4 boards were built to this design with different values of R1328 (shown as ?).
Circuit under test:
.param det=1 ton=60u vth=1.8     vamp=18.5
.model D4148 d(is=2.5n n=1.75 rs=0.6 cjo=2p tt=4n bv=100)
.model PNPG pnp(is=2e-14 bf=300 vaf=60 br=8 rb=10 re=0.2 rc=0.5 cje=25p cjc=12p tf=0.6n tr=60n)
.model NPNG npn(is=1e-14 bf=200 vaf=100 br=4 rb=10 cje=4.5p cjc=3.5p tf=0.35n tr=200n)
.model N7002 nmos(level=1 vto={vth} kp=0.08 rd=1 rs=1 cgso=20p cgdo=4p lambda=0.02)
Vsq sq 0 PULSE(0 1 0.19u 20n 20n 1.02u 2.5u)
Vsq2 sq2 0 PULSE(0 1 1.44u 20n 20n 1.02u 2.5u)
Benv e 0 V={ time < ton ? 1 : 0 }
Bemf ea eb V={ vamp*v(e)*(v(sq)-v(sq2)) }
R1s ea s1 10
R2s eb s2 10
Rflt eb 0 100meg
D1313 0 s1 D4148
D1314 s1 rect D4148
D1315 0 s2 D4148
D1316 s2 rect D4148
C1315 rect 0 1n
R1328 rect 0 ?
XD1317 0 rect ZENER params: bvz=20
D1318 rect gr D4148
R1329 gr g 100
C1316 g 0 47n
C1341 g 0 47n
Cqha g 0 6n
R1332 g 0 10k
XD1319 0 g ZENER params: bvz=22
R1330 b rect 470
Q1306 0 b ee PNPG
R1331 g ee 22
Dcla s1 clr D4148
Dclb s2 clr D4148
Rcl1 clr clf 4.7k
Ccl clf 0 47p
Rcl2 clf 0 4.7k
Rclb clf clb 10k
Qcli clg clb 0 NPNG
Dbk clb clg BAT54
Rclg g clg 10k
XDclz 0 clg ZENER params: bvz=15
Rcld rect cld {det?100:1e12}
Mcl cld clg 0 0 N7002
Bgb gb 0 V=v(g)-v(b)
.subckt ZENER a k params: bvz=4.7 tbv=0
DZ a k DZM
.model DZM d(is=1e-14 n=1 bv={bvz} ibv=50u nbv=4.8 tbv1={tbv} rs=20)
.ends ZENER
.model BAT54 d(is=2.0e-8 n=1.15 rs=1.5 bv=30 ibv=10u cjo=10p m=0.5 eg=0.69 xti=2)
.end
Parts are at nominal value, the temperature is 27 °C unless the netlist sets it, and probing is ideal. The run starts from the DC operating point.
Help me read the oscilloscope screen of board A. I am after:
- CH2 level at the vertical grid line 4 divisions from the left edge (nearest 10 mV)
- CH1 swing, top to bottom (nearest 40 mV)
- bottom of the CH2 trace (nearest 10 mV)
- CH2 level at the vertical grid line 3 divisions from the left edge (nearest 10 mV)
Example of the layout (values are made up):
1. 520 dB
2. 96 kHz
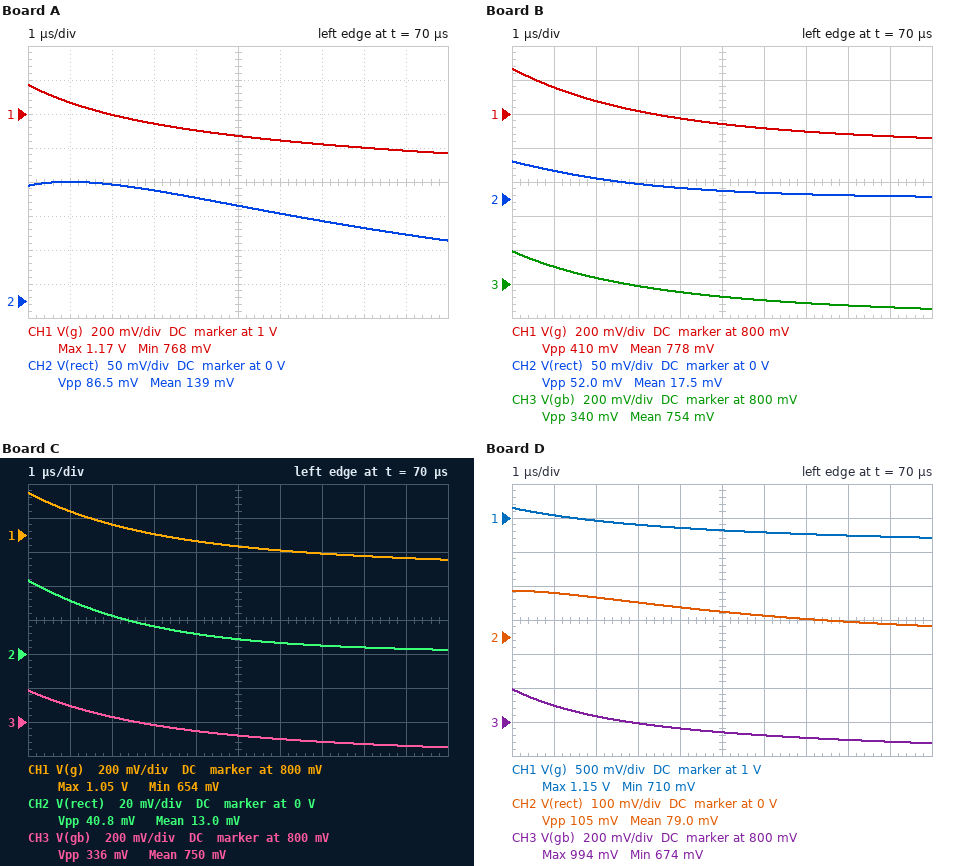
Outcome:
1. 150 mV
2. 400 mV
3. 90 mV
4. 160 mV
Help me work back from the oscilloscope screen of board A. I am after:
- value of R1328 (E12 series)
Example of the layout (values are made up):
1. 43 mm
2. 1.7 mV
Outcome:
1. 6.8 kΩ
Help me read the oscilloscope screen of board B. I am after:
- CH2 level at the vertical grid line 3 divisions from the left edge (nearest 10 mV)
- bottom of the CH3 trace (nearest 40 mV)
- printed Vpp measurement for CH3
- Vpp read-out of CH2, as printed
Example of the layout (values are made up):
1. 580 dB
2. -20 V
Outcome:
1. 20 mV
2. 640 mV
3. 340 mV
4. 52.0 mV
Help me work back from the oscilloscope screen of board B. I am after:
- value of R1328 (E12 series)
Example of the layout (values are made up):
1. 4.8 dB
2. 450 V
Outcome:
1. 1 kΩ
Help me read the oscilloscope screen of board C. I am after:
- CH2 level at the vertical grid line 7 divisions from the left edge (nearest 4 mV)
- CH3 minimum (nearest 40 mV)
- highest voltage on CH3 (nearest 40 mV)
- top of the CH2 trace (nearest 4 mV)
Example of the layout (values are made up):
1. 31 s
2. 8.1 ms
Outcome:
1. 4 mV
2. 640 mV
3. 1.00 V
4. 44 mV
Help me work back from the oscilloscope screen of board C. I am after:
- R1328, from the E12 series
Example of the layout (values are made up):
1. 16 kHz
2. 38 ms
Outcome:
1. 820 Ω
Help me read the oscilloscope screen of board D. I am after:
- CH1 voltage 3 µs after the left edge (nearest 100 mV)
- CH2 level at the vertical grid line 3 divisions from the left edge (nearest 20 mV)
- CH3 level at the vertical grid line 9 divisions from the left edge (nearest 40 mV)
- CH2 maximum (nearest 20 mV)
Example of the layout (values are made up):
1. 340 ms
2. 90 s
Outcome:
1. 900 mV
2. 100 mV
3. 680 mV
4. 140 mV
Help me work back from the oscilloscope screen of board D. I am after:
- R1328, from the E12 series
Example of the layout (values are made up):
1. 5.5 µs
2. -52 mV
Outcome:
1. 3.3 kΩ
